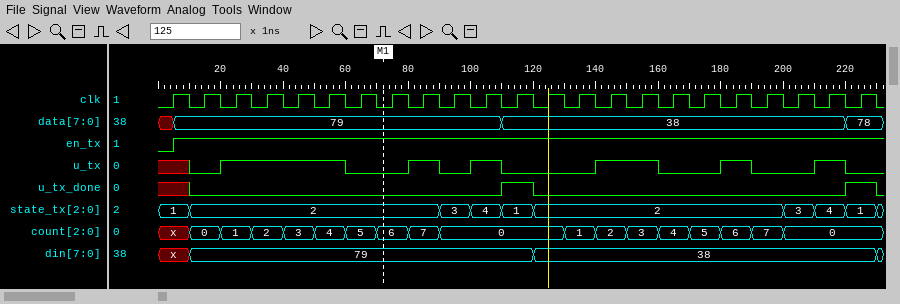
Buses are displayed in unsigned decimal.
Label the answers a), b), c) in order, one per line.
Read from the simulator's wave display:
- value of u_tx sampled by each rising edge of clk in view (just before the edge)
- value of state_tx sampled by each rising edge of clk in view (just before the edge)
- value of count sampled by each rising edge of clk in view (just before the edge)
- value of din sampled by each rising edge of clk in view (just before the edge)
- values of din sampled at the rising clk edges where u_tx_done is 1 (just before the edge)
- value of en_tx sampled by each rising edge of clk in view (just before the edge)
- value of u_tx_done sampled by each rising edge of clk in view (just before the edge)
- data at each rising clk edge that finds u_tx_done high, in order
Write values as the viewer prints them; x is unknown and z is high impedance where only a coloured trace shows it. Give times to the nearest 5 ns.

a) x 0 1 1 1 1 0 0 1 0 1 0 0 0 1 1 0 0 1 0 0 1 0
b) 1, 2, 2, 2, 2, 2, 2, 2, 2, 3, 4, 1, 2, 2, 2, 2, 2, 2, 2, 2, 3, 4, 1
c) x, 0, 1, 2, 3, 4, 5, 6, 7, 0, 0, 0, 0, 1, 2, 3, 4, 5, 6, 7, 0, 0, 0
d) x, 79, 79, 79, 79, 79, 79, 79, 79, 79, 79, 79, 38, 38, 38, 38, 38, 38, 38, 38, 38, 38, 38
e) 79, 38
f) 0 1 1 1 1 1 1 1 1 1 1 1 1 1 1 1 1 1 1 1 1 1 1
g) x 0 0 0 0 0 0 0 0 0 0 1 0 0 0 0 0 0 0 0 0 0 1
h) 38, 78
